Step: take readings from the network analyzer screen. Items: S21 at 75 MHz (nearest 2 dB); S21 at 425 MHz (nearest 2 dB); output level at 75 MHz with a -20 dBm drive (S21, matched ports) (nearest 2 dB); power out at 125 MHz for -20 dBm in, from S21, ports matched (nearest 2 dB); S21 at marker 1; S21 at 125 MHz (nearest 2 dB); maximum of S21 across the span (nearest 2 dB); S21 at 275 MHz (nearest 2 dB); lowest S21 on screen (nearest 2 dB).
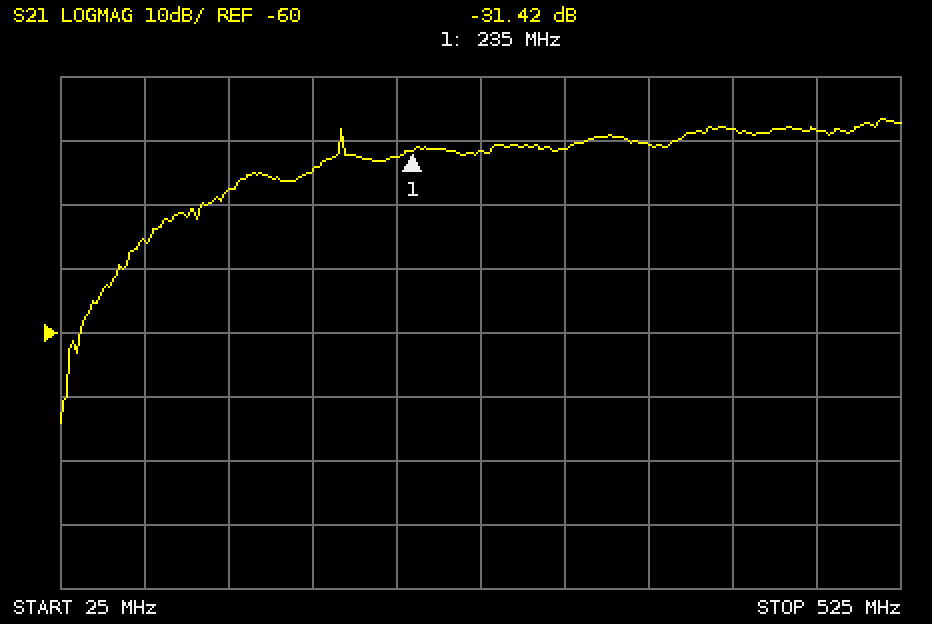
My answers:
-46 dB
-28 dB
-66 dBm
-58 dBm
-31.42 dB
-38 dB
-26 dB
-32 dB
-74 dB
